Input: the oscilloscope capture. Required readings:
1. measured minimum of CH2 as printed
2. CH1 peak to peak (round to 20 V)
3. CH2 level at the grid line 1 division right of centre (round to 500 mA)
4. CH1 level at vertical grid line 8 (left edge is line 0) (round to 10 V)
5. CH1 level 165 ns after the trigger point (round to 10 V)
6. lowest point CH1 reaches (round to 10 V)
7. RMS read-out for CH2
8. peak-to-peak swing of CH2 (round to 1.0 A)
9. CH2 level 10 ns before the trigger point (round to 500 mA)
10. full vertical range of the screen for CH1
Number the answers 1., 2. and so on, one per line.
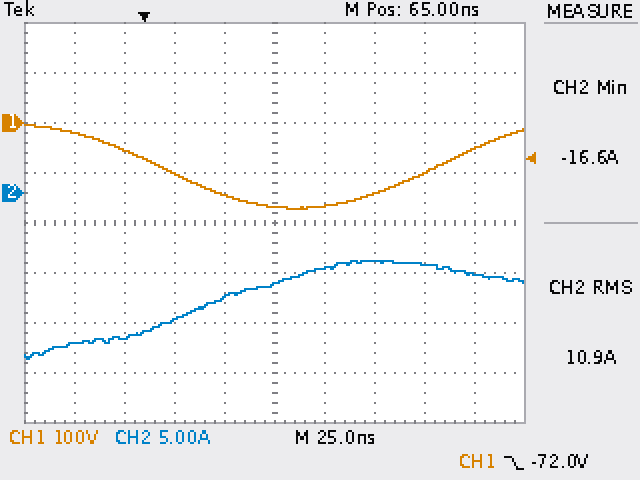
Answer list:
1. -16.6 A
2. 160 V
3. -7.5 A
4. -100 V
5. -50 V
6. -170 V
7. 10.9 A
8. 10.0 A
9. -14.5 A
10. 800 V
